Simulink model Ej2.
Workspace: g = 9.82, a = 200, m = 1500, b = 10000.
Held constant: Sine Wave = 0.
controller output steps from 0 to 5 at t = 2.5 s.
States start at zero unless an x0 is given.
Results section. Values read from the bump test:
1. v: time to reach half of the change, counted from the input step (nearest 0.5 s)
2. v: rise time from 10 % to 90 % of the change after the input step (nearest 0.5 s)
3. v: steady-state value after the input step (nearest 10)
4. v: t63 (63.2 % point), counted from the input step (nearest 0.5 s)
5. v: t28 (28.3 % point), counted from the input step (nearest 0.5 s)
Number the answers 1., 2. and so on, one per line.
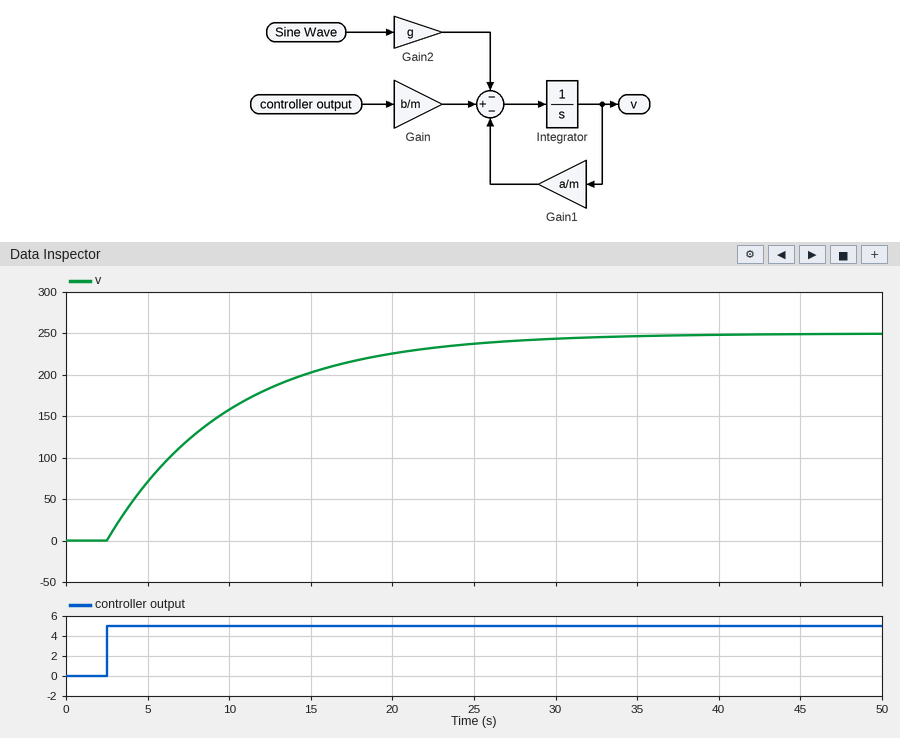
1. 5.0 s
2. 16.5 s
3. 250
4. 7.5 s
5. 2.5 s
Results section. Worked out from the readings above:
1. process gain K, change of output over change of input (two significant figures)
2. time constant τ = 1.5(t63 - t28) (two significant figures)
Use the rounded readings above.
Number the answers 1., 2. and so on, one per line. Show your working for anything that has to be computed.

1. (250 - 0) / 5 = 50
2. 1.5 × (7.5 - 2.5) = 7.5 s
